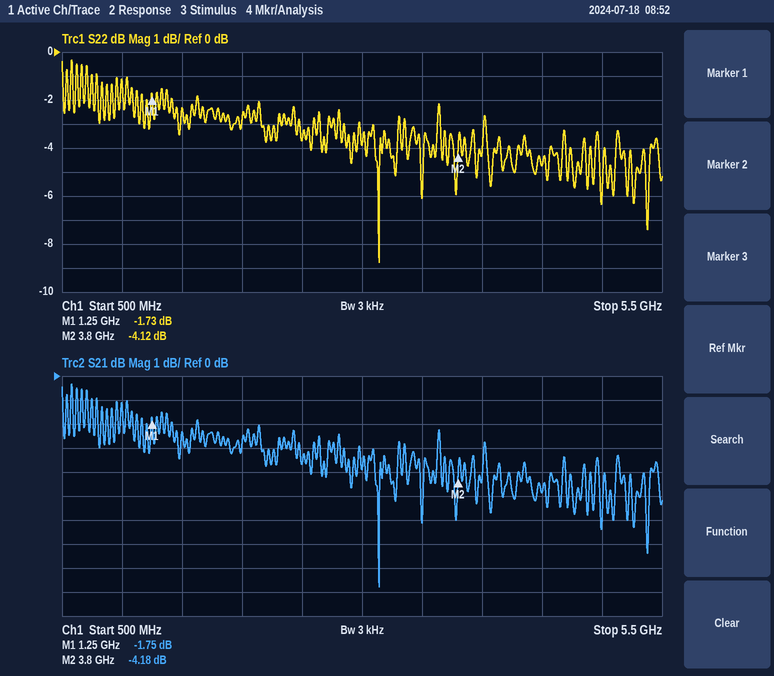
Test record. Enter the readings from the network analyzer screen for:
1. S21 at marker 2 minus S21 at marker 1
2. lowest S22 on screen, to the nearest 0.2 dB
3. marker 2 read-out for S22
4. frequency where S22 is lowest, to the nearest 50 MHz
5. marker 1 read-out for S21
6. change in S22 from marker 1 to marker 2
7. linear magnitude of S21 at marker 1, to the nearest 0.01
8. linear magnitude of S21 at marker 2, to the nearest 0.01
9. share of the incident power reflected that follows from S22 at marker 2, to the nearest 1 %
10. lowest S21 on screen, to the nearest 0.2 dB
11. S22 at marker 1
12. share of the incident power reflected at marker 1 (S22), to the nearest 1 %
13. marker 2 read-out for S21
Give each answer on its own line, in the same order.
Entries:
-2.43 dB
-8.8 dB
-4.12 dB
3.15 GHz
-1.75 dB
-2.39 dB
0.82
0.62
39 %
-8.8 dB
-1.73 dB
67 %
-4.18 dB
